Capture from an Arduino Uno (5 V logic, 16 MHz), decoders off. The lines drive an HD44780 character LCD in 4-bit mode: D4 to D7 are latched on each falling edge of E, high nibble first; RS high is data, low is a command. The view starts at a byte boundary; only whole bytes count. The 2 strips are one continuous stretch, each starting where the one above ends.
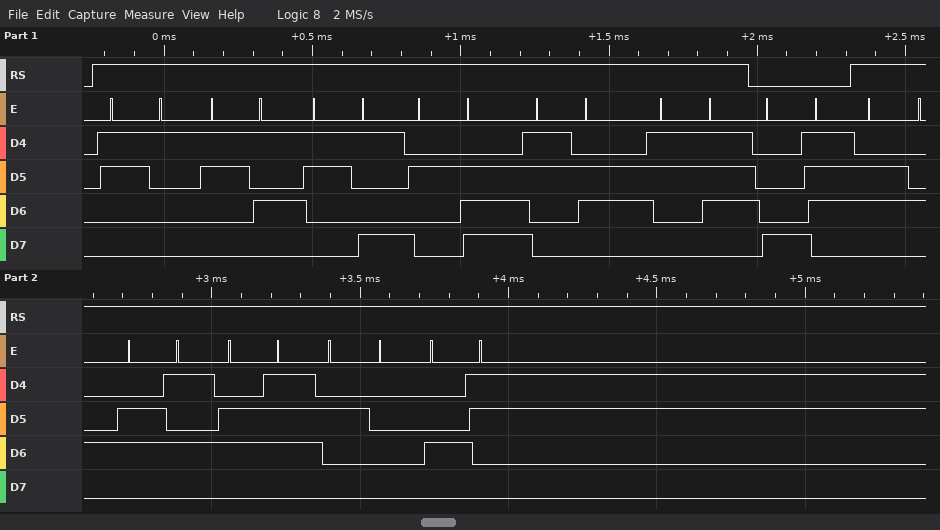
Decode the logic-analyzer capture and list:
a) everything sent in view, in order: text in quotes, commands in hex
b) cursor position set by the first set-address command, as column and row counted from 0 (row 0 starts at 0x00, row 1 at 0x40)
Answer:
"159.67" 0x87 "deg C"
column 7, row 0
